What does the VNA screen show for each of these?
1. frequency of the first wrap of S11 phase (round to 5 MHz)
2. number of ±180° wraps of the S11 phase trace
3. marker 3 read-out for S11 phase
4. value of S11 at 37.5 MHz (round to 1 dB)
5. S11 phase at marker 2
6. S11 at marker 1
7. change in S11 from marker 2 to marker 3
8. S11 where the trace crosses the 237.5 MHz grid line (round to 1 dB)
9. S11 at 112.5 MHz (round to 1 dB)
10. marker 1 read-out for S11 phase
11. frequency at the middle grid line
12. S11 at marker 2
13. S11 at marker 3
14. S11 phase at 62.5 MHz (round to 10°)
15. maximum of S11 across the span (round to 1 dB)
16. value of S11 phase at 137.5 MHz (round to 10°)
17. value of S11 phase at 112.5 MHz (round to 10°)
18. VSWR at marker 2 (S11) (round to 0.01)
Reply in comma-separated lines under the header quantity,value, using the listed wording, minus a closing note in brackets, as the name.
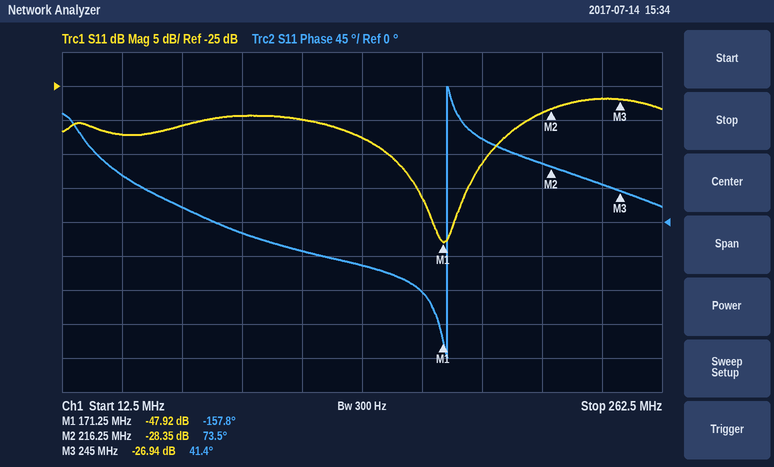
quantity,value
frequency of the first wrap of S11 phase,175 MHz
number of ±180° wraps of the S11 phase trace,1
marker 3 read-out for S11 phase,41.4°
value of S11 at 37.5 MHz,-32 dB
S11 phase at marker 2,73.5°
S11 at marker 1,-47.92 dB
change in S11 from marker 2 to marker 3,1.41 dB
S11 where the trace crosses the 237.5 MHz grid line,-27 dB
S11 at 112.5 MHz,-30 dB
marker 1 read-out for S11 phase,-157.8°
frequency at the middle grid line,137.5 MHz
S11 at marker 2,-28.35 dB
S11 at marker 3,-26.94 dB
S11 phase at 62.5 MHz,20°
maximum of S11 across the span,-27 dB
value of S11 phase at 137.5 MHz,-60°
value of S11 phase at 112.5 MHz,-40°
VSWR at marker 2 (S11),1.08
